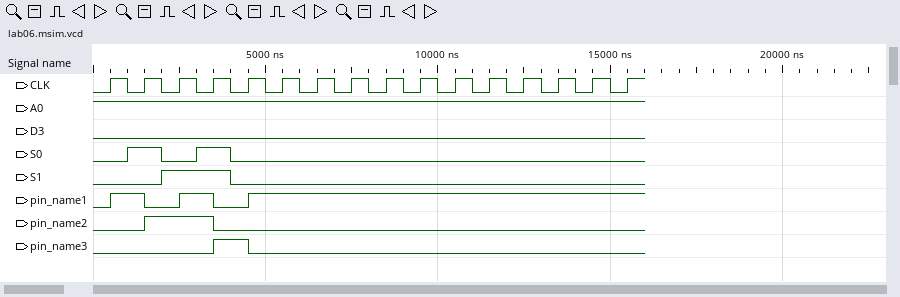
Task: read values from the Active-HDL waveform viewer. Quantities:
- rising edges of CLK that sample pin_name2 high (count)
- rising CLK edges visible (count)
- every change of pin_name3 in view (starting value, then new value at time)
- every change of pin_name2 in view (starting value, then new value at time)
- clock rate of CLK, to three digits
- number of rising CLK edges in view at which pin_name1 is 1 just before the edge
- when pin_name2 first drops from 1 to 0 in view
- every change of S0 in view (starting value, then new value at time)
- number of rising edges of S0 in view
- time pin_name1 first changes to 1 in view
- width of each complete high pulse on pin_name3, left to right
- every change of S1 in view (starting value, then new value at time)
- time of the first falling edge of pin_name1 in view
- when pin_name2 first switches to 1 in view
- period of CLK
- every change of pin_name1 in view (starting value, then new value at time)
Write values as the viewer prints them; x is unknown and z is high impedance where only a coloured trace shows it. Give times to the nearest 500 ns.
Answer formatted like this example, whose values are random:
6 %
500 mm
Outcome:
2
16
0, 1 at 3500 ns, 0 at 4500 ns
0, 1 at 1500 ns, 0 at 3500 ns
1.00 MHz
13
3500 ns
0, 1 at 1000 ns, 0 at 2000 ns, 1 at 3000 ns, 0 at 4000 ns
2
500 ns
1000 ns
0, 1 at 2000 ns, 0 at 4000 ns
1500 ns
1500 ns
1000 ns
0, 1 at 500 ns, 0 at 1500 ns, 1 at 2500 ns, 0 at 3500 ns, 1 at 4500 ns
